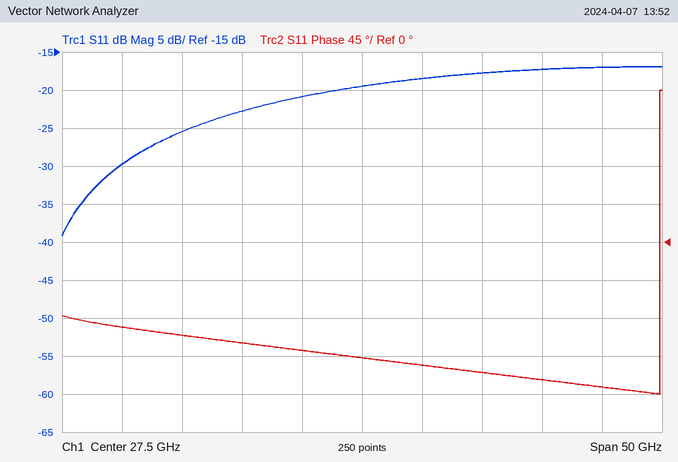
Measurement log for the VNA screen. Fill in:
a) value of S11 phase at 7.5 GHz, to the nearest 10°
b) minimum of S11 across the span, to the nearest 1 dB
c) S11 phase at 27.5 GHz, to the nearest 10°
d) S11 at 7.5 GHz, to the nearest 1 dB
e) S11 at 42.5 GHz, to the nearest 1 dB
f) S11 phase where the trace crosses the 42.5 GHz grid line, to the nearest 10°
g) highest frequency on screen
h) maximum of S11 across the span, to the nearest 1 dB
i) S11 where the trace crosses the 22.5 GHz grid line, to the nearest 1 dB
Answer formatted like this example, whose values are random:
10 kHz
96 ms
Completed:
-100°
-39 dB
-140°
-30 dB
-17 dB
-160°
52.5 GHz
-17 dB
-21 dB
